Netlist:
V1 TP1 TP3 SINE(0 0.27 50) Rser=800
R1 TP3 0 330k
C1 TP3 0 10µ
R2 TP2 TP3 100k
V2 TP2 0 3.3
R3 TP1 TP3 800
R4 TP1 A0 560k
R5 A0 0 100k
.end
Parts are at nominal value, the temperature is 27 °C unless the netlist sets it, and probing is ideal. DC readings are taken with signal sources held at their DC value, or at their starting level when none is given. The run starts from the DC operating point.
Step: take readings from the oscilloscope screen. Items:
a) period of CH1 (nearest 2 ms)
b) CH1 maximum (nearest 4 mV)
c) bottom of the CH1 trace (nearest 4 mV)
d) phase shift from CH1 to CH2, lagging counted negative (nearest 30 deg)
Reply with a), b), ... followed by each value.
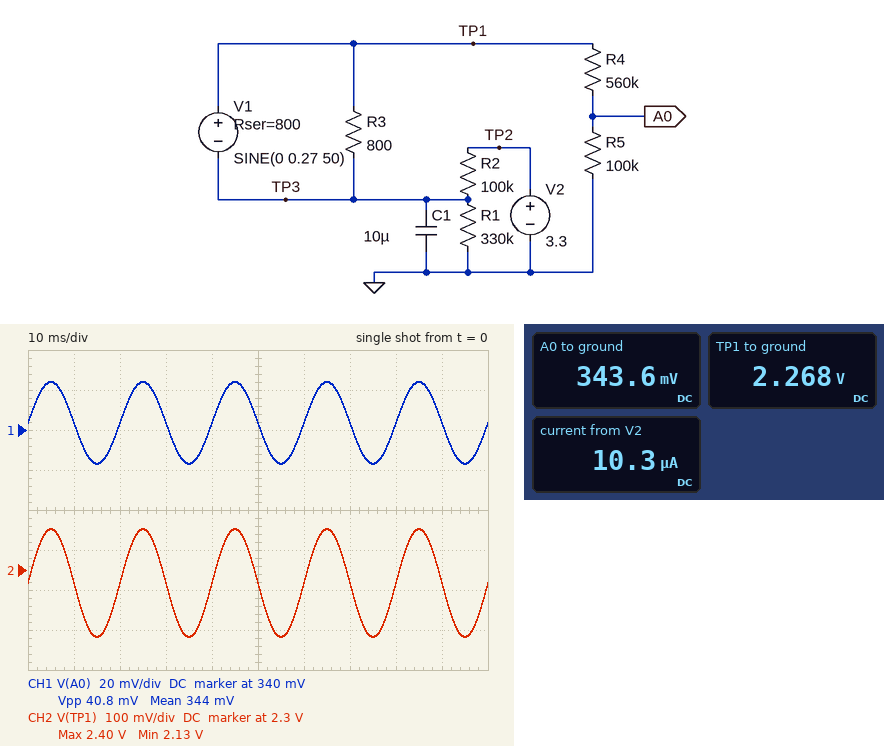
a) 20 ms
b) 364 mV
c) 324 mV
d) 0 deg
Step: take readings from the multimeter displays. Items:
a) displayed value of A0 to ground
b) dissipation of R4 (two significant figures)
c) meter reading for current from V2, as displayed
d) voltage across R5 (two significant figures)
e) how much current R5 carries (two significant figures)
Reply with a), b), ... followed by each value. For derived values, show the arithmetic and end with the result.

a) 343.6 mV
b) (2.268 V - 343.6 mV)^2 / 560 kΩ = 6.6 µW
c) 10.3 µA
d) 343.6 mV = 340 mV
e) (343.6 mV) / 100 kΩ = 3.4 µA
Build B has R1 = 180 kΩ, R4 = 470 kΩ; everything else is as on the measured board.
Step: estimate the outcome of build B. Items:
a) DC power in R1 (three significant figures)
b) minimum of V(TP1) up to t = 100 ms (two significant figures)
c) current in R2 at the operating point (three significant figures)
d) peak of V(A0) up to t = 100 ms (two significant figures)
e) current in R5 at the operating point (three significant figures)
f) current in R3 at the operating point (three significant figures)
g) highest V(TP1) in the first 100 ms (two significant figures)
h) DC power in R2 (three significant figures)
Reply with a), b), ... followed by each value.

a) 20.2 µW
b) 1.8 V
c) 13.9 µA
d) 360 mV
e) 3.34 µA
f) 1.67 µA
g) 2.0 V
h) 19.4 µW
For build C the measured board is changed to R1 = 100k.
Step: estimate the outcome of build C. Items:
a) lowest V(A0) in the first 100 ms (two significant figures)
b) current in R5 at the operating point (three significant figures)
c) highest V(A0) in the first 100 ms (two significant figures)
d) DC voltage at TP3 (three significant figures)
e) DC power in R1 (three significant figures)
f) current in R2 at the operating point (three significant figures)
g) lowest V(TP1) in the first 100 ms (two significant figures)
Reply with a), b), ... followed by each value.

a) 210 mV
b) 2.32 µA
c) 250 mV
d) 1.53 V
e) 23.5 µW
f) 17.7 µA
g) 1.4 V
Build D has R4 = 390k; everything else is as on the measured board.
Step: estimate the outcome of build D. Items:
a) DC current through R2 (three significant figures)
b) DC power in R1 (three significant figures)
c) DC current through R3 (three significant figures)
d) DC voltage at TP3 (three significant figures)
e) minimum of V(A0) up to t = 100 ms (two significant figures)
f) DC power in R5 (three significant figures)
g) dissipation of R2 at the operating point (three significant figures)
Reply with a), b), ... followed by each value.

a) 11.1 µA
b) 14.5 µW
c) 2.23 µA
d) 2.19 V
e) 420 mV
f) 1.99 µW
g) 12.3 µW
